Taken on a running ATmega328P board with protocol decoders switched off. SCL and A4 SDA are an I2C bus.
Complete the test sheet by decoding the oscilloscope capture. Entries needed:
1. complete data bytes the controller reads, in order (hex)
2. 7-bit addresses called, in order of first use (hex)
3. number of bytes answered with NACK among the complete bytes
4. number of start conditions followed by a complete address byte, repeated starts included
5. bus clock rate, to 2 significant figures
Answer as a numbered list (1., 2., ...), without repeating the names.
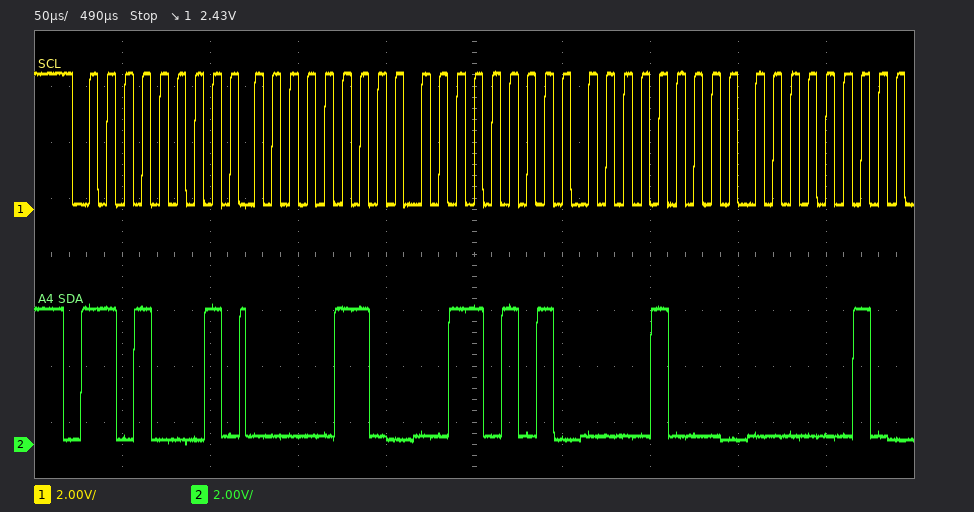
1. 06 35 08 02
2. 0x68
3. 0
4. 1
5. 100 kHz
